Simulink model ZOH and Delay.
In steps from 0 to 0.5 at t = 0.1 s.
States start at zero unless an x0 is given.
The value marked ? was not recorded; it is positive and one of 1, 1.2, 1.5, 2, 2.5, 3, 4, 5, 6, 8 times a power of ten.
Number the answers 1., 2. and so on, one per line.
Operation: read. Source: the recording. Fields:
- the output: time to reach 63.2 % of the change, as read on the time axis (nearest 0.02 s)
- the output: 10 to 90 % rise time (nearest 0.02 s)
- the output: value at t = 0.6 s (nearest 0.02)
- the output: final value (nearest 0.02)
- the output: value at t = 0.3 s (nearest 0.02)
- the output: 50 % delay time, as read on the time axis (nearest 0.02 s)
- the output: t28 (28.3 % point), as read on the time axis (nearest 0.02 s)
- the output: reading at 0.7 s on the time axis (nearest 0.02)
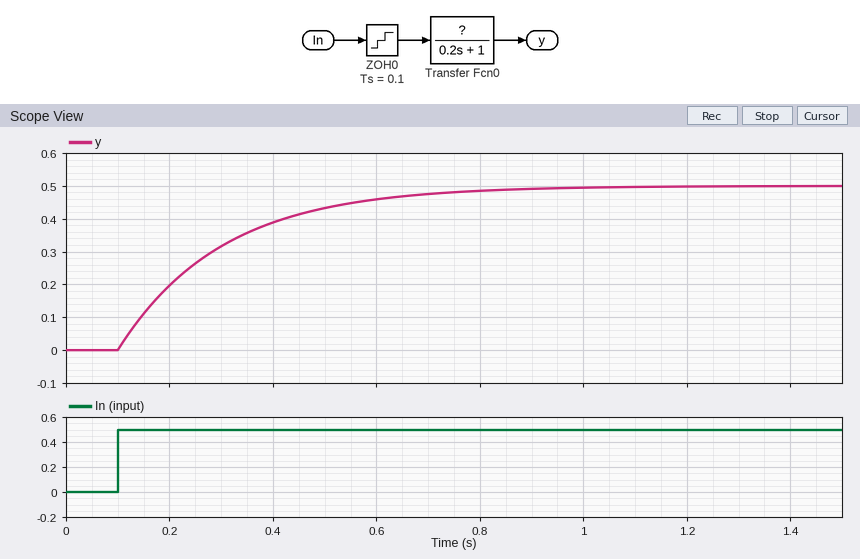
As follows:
1. 0.30 s
2. 0.44 s
3. 0.46
4. 0.50
5. 0.32
6. 0.24 s
7. 0.16 s
8. 0.48
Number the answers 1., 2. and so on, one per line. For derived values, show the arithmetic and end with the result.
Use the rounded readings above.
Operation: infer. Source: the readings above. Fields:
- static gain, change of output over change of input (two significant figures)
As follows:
1. (0.5 - 0) / (0.5 - 0) = 1.0
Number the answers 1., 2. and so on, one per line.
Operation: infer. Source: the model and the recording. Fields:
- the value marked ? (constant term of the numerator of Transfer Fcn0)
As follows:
1. 1
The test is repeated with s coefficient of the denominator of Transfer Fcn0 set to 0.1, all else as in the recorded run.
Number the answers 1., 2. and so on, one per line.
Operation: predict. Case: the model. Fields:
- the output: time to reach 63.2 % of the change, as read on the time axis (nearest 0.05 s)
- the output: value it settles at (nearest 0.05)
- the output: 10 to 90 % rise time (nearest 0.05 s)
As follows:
1. 0.20 s
2. 0.50
3. 0.20 s
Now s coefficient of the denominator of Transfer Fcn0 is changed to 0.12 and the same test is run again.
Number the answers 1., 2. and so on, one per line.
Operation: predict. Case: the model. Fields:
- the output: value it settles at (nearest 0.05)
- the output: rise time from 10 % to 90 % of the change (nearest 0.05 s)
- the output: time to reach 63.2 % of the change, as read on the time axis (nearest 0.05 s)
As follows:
1. 0.50
2. 0.25 s
3. 0.20 s
